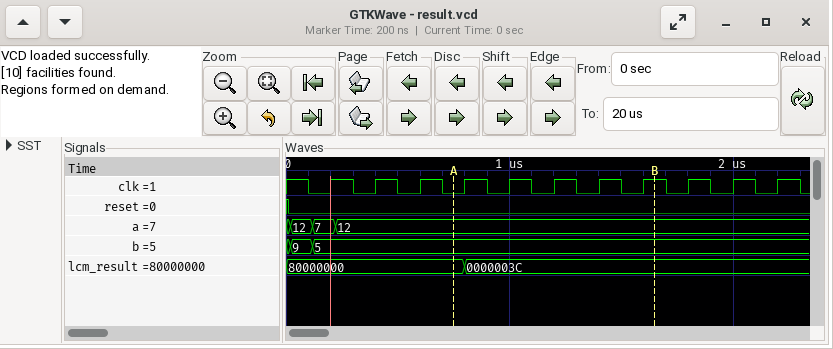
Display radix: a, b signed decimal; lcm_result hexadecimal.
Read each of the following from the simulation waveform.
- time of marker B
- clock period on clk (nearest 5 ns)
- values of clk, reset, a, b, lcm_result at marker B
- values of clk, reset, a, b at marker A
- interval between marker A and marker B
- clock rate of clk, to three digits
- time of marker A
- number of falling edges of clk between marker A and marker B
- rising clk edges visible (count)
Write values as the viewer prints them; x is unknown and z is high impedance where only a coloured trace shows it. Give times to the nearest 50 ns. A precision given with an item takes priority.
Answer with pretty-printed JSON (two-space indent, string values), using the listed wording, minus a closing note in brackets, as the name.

{
  "time of marker B": "1650 ns",
  "clock period on clk": "200 ns",
  "values of clk, reset, a, b, lcm_result at marker B": "clk=1, reset=0, a=12, b=5, lcm_result=0000003C",
  "values of clk, reset, a, b at marker A": "clk=0, reset=0, a=12, b=5",
  "interval between marker A and marker B": "900 ns",
  "clock rate of clk, to three digits": "5.00 MHz",
  "time of marker A": "750 ns",
  "number of falling edges of clk between marker A and marker B": "4",
  "rising clk edges visible": "11"
}
